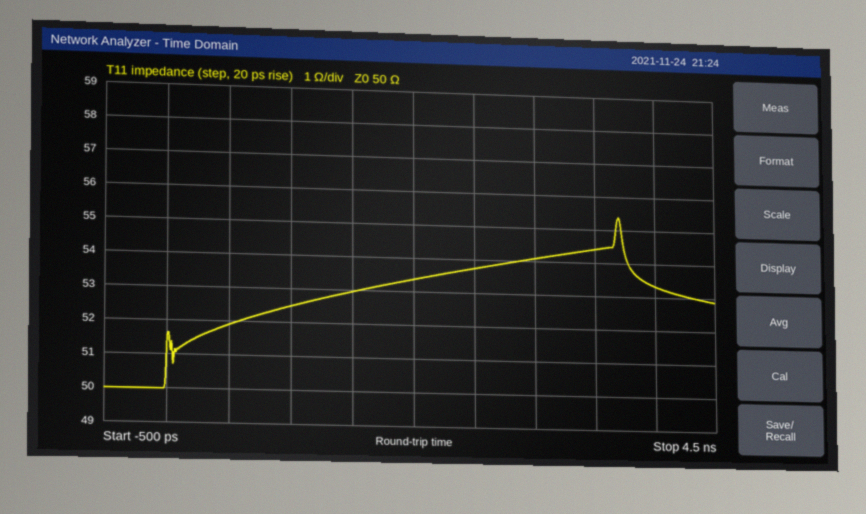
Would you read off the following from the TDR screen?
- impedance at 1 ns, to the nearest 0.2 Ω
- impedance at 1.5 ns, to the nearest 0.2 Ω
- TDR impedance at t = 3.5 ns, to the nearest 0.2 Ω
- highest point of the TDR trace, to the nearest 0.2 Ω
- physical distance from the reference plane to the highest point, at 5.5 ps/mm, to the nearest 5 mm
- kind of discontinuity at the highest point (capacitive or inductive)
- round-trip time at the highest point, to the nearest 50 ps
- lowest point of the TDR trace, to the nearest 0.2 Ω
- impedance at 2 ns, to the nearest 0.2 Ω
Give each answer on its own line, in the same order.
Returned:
52.4 Ω
53.0 Ω
54.4 Ω
55.4 Ω
335 mm
inductive
3.70 ns
50.0 Ω
53.4 Ω
